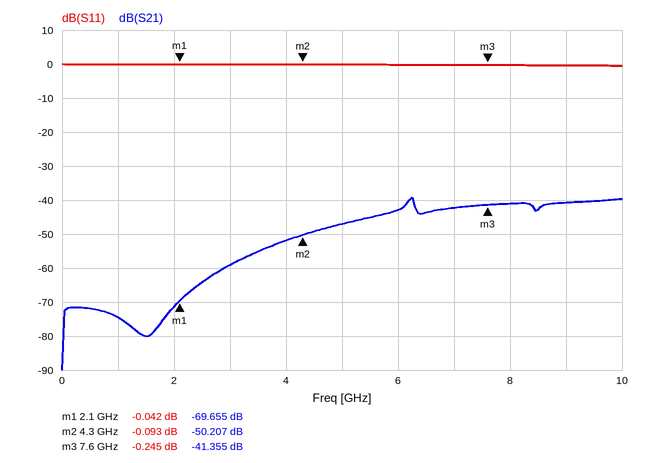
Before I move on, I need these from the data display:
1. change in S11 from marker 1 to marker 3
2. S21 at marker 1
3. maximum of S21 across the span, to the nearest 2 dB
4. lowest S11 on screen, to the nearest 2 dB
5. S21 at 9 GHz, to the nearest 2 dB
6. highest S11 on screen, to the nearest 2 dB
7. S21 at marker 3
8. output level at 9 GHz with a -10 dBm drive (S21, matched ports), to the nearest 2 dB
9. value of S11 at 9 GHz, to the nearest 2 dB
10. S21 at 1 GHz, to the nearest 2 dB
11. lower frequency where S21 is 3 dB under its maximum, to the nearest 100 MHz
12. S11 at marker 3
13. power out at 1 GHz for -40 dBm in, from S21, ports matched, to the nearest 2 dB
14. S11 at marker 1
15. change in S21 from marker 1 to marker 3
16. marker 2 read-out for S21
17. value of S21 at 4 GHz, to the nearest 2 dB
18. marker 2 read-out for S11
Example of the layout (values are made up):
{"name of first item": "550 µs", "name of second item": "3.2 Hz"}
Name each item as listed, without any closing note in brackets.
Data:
{"change in S11 from marker 1 to marker 3": "-0.203 dB", "S21 at marker 1": "-69.655 dB", "maximum of S21 across the span, to the nearest 2 dB": "-40 dB", "lowest S11 on screen, to the nearest 2 dB": "0 dB", "S21 at 9 GHz, to the nearest 2 dB": "-40 dB", "highest S11 on screen, to the nearest 2 dB": "0 dB", "S21 at marker 3": "-41.355 dB", "output level at 9 GHz with a -10 dBm drive (S21, matched ports), to the nearest 2 dB": "-50 dBm", "value of S11 at 9 GHz, to the nearest 2 dB": "0 dB", "S21 at 1 GHz, to the nearest 2 dB": "-74 dB", "lower frequency where S21 is 3 dB under its maximum, to the nearest 100 MHz": "6.1 GHz", "S11 at marker 3": "-0.245 dB", "power out at 1 GHz for -40 dBm in, from S21, ports matched, to the nearest 2 dB": "-114 dBm", "S11 at marker 1": "-0.042 dB", "change in S21 from marker 1 to marker 3": "28.300 dB", "marker 2 read-out for S21": "-50.207 dB", "value of S21 at 4 GHz, to the nearest 2 dB": "-52 dB", "marker 2 read-out for S11": "-0.093 dB"}
